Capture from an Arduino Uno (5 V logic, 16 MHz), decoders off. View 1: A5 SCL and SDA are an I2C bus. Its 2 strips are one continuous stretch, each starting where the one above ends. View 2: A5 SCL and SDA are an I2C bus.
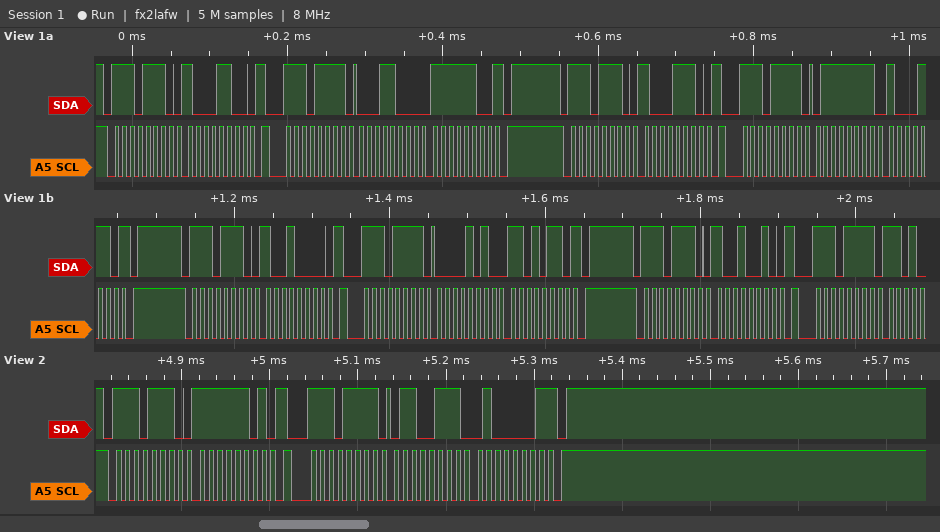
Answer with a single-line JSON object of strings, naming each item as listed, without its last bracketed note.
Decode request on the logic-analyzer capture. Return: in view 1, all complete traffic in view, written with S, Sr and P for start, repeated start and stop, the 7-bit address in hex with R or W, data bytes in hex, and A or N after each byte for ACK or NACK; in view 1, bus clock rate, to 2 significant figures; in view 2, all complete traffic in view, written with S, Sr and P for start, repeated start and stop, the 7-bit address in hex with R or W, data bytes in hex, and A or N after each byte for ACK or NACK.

{"in view 1, all complete traffic in view, written with S, Sr and P for start, repeated start and stop, the 7-bit address in hex with R or W, data bytes in hex, and A or N after each byte for ACK or NACK": "S 77W A 8C A Sr 77R A 18 A FC N P S 77W A 8E A Sr 77R A 7F A 8E N P S 77W A 90 A Sr 77R A 0A A D6 N P S 77W A 92 A Sr 77R A", "in view 1, bus clock rate, to 2 significant figures": "100 kHz", "in view 2, all complete traffic in view, written with S, Sr and P for start, repeated start and stop, the 7-bit address in hex with R or W, data bytes in hex, and A or N after each byte for ACK or NACK": "S 77W A FD A Sr 77R A 67 A 41 N P"}
